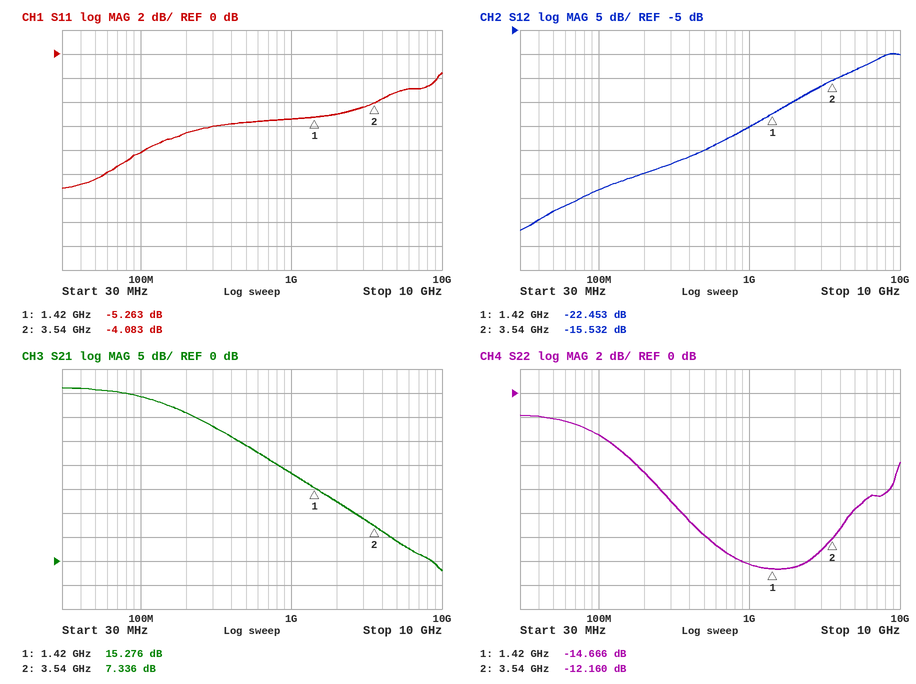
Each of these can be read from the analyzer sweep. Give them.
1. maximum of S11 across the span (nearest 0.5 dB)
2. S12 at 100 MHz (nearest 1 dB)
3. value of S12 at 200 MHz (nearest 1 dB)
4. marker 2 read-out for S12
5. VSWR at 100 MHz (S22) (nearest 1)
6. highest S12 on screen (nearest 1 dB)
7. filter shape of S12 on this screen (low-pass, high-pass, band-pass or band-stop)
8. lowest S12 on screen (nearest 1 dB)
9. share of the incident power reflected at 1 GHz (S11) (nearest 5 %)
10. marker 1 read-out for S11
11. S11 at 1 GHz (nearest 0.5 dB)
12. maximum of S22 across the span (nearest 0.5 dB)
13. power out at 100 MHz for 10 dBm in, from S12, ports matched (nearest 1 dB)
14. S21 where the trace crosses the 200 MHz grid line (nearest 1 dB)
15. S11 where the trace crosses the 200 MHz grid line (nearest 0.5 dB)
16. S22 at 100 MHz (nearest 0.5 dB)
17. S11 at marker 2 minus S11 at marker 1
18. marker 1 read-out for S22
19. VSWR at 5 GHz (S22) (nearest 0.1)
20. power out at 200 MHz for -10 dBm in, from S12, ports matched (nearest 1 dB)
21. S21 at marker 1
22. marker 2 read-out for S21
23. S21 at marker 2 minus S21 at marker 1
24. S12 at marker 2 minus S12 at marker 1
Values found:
-1.5 dB
-38 dB
-35 dB
-15.532 dB
5
-10 dB
high-pass
-47 dB
30 %
-5.263 dB
-5.5 dB
-2.0 dB
-28 dBm
31 dB
-6.5 dB
-3.5 dB
1.180 dB
-14.666 dB
2.0
-45 dBm
15.276 dB
7.336 dB
-7.940 dB
6.921 dB
